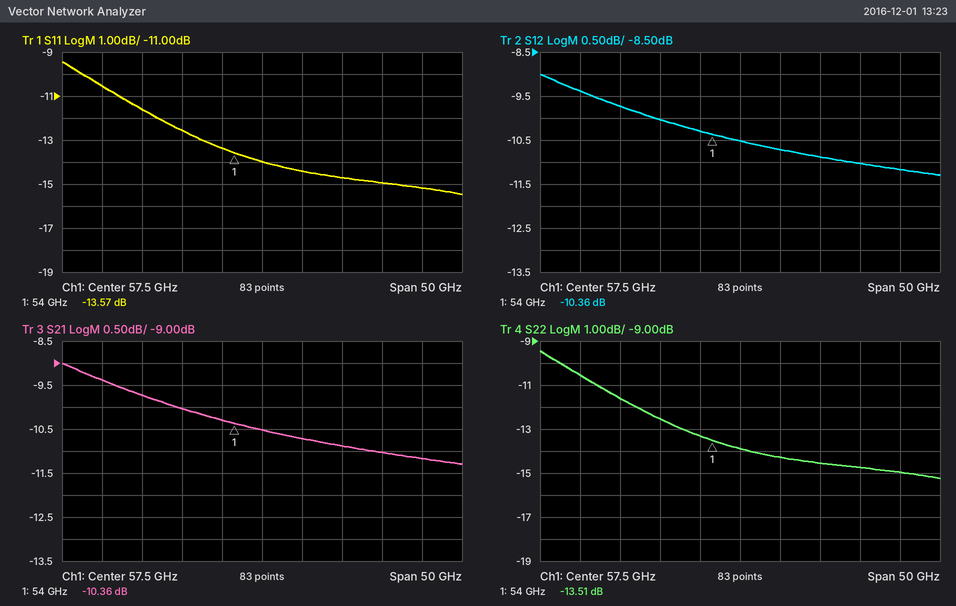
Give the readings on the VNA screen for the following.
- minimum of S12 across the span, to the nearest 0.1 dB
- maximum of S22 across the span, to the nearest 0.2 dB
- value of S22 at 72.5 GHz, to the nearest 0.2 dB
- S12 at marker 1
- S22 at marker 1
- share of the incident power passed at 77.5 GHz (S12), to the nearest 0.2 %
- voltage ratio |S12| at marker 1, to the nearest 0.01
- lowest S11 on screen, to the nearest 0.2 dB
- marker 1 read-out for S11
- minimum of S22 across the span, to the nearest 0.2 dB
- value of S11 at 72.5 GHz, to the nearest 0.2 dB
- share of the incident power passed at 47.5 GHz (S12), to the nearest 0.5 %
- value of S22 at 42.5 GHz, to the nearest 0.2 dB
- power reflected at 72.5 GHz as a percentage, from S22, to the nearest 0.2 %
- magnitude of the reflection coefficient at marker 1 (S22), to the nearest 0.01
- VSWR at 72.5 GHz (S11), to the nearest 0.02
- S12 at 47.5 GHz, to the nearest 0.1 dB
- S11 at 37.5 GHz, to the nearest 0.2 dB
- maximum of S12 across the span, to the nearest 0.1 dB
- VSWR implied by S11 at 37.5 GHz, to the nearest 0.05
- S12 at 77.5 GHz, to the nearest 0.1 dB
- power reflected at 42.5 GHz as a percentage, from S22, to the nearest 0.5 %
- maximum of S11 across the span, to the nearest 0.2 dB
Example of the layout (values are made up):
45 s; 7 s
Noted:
-11.3 dB; -9.4 dB; -14.8 dB; -10.36 dB; -13.51 dB; 7.6 %; 0.30; -15.4 dB; -13.57 dB; -15.2 dB; -15.0 dB; 10.0 %; -11.6 dB; 3.4 %; 0.21; 1.44; -10.0 dB; -10.6 dB; -9.0 dB; 1.85; -11.2 dB; 7.0 %; -9.4 dB
